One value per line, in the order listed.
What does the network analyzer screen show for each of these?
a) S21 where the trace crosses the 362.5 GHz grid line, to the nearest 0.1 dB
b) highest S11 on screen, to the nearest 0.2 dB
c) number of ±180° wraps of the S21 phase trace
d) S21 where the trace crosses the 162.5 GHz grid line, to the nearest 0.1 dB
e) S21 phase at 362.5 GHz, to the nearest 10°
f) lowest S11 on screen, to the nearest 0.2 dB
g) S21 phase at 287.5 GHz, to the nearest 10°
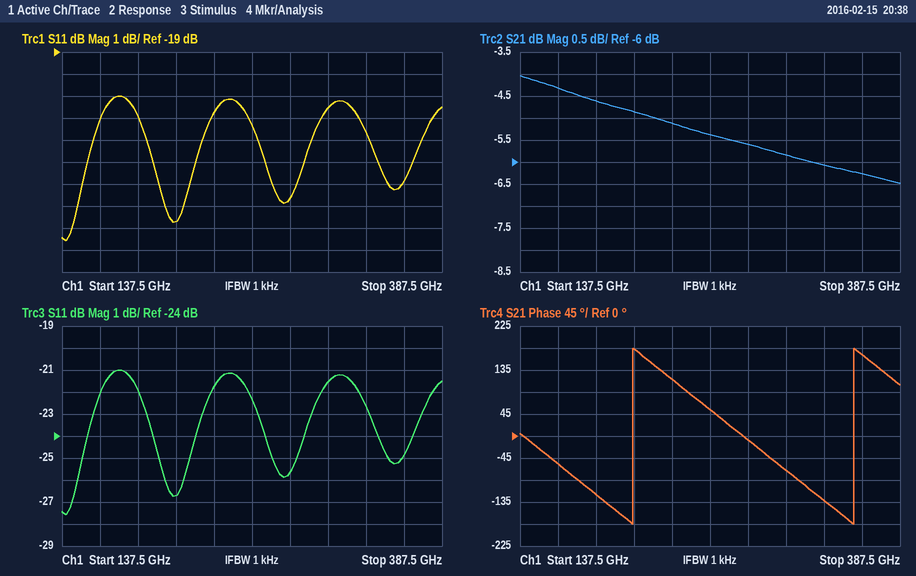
-6.3 dB
-21.0 dB
2
-4.3 dB
170°
-27.6 dB
-10°
